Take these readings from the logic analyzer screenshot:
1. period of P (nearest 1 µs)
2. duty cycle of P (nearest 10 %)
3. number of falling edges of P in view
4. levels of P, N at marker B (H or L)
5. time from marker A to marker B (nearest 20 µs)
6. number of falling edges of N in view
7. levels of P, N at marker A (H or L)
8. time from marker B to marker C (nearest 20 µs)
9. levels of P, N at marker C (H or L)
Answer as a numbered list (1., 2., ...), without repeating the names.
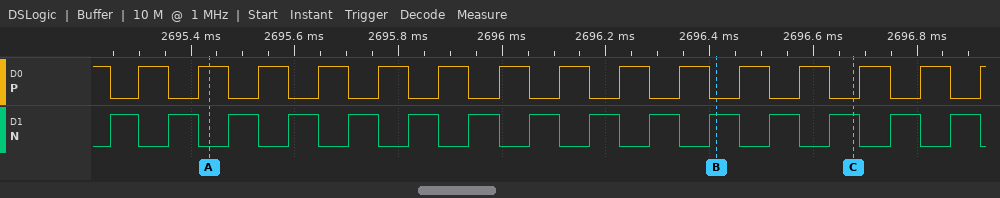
1. 116 µs
2. 50 %
3. 15
4. P=L, N=H
5. 980 µs
6. 15
7. P=H, N=L
8. 260 µs
9. P=L, N=H
